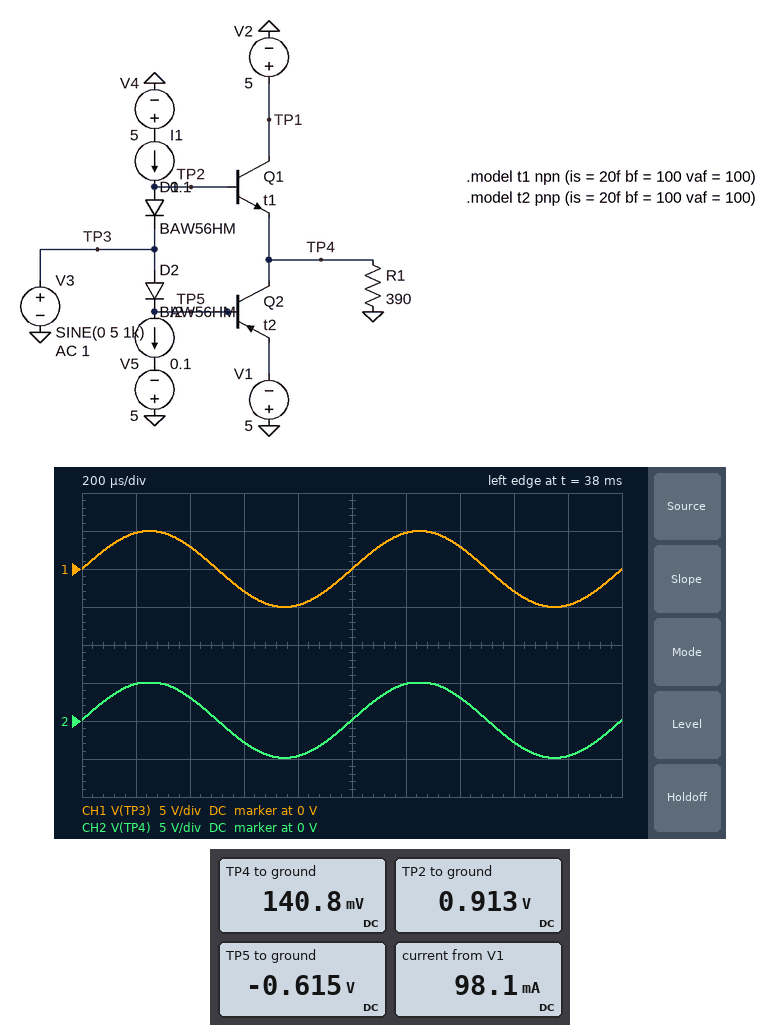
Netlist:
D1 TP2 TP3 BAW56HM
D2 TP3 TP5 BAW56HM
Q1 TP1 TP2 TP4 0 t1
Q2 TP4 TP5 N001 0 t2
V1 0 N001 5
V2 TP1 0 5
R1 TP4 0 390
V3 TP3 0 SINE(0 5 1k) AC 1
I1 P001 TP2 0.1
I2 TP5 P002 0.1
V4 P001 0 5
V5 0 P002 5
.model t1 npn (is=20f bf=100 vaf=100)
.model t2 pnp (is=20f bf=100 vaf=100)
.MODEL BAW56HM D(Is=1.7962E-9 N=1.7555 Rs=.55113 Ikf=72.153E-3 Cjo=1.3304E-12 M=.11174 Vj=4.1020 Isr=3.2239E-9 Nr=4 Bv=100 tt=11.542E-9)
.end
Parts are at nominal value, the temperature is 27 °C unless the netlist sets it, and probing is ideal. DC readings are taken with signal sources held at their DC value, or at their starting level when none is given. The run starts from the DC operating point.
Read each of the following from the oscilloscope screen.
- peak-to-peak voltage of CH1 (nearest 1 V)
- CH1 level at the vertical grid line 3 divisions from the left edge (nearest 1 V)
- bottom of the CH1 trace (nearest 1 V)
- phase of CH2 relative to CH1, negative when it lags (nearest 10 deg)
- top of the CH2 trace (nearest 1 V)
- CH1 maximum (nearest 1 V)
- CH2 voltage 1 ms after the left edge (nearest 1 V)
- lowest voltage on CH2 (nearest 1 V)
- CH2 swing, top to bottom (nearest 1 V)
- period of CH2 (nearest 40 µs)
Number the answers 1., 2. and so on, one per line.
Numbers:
1. 10 V
2. -3 V
3. -5 V
4. 0 deg
5. 5 V
6. 5 V
7. 0 V
8. -5 V
9. 10 V
10. 1.00 ms
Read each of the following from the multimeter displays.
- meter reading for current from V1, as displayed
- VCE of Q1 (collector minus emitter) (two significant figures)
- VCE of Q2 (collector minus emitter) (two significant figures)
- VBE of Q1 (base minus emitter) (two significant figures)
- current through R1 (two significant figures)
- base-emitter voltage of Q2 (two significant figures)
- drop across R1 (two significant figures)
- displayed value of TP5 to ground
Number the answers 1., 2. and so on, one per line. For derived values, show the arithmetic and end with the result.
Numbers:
1. 98.1 mA
2. 5 V - 140.8 mV = 4.9 V
3. 140.8 mV - (-5 V) = 5.1 V
4. 913 mV - 140.8 mV = 770 mV
5. (140.8 mV) / 390 Ω = 360 µA
6. -615 mV - (-5 V) = 4.4 V
7. 140.8 mV = 140 mV
8. -0.615 V
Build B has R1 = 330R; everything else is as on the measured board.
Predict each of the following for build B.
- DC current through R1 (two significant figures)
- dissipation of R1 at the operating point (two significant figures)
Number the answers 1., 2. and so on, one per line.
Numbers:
1. 430 µA
2. 60 µW
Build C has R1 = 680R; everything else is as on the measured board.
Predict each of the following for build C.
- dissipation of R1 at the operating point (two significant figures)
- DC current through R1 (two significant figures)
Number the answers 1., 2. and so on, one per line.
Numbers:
1. 29 µW
2. 210 µA
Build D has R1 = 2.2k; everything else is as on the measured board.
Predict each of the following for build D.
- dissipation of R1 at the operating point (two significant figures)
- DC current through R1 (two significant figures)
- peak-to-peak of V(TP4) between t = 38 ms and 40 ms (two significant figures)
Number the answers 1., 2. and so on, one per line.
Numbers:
1. 9.0 µW
2. 64 µA
3. 9.8 V
